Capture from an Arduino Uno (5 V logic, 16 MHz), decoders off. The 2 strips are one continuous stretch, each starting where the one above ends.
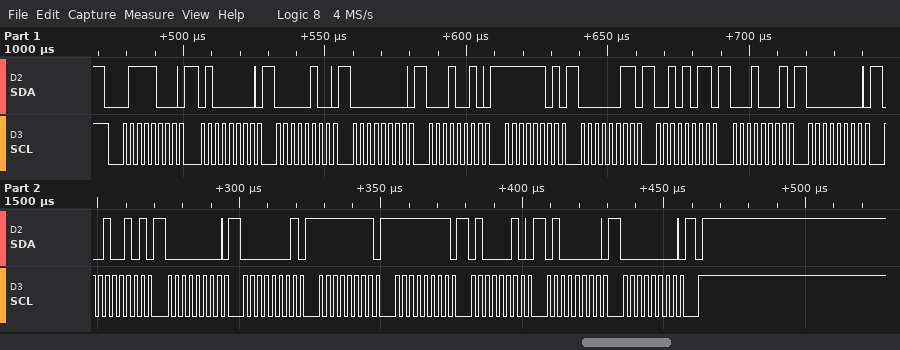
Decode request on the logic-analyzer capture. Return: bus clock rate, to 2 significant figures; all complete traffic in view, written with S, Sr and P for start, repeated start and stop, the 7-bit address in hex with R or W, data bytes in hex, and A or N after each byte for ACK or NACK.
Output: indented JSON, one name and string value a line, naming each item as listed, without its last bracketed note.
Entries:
{
  "bus clock rate, to 2 significant figures": "400 kHz",
  "all complete traffic in view, written with S, Sr and P for start, repeated start and stop, the 7-bit address in hex with R or W, data bytes in hex, and A or N after each byte for ACK or NACK": "S 3CW A 40 A 04 A 00 A 12 A FD A 03 A 2B A 11 A 00 A 25 A 00 A 01 A FF A FF A 42 A 40 A 00 A P"
}
